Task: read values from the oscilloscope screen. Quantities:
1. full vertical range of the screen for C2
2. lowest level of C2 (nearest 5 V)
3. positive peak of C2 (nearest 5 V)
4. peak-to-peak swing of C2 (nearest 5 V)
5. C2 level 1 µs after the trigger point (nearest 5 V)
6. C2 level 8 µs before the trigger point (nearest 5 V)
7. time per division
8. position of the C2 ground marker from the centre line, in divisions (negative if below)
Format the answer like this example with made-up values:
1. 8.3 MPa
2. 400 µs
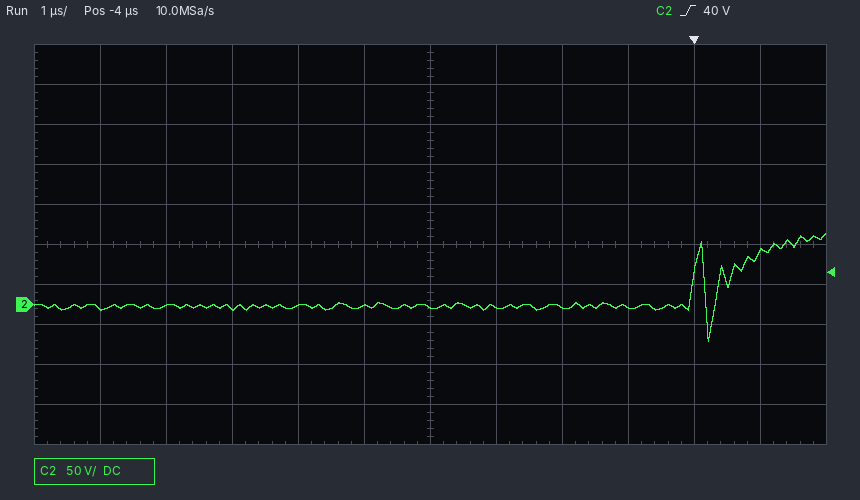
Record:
1. 500 V
2. -45 V
3. 90 V
4. 135 V
5. 65 V
6. 0 V
7. 1 µs
8. -1.5 div
